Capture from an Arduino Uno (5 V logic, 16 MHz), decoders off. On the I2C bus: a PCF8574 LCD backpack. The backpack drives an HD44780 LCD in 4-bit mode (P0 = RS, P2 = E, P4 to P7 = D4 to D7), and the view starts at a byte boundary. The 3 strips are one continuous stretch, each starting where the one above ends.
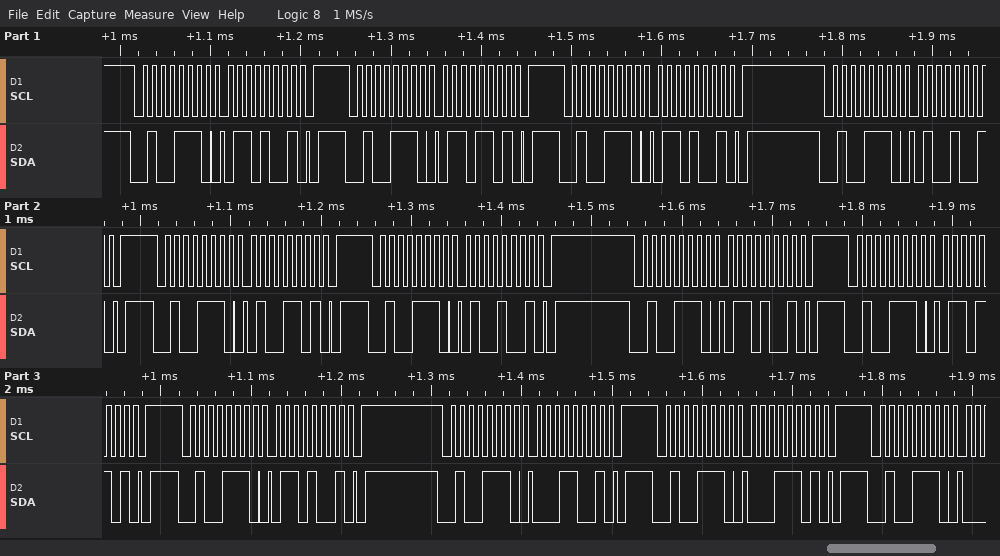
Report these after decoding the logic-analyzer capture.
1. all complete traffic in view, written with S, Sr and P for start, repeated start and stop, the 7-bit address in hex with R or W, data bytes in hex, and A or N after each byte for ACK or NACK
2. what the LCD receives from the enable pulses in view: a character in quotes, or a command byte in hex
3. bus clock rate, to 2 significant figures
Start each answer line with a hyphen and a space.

- S 27W A 69 A P S 27W A 6D A P S 27W A 69 A P S 27W A 49 A P S 27W A 4D A P S 27W A 49 A P S 27W A 69 A P S 27W A 6D A P S 27W A 69 A P S 27W A 19 A P S 27W A 1D A P S 27W A
- 'd'
- 100 kHz
